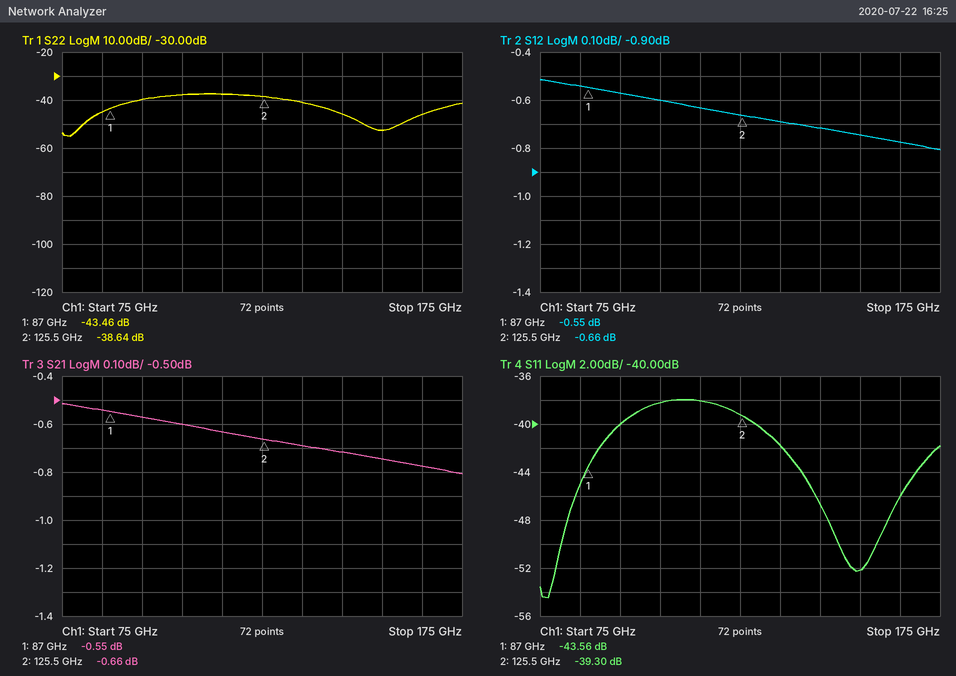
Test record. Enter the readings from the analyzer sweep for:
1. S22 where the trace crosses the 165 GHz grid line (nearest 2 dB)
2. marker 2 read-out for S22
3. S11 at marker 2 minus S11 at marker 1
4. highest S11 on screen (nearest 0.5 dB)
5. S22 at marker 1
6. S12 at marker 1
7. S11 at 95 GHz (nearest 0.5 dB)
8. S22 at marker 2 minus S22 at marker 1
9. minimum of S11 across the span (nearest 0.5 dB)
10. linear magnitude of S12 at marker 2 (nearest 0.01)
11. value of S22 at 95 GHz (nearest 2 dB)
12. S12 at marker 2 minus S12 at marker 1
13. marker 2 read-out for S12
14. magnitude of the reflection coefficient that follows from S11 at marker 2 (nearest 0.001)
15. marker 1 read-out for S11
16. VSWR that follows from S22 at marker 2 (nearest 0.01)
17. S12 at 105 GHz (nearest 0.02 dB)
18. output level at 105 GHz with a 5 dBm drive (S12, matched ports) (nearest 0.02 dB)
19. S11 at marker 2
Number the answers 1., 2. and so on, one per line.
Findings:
1. -46 dB
2. -38.64 dB
3. 4.26 dB
4. -38.0 dB
5. -43.46 dB
6. -0.55 dB
7. -40.0 dB
8. 4.82 dB
9. -54.5 dB
10. 0.93
11. -40 dB
12. -0.11 dB
13. -0.66 dB
14. 0.011
15. -43.56 dB
16. 1.02
17. -0.60 dB
18. 4.40 dBm
19. -39.30 dB
